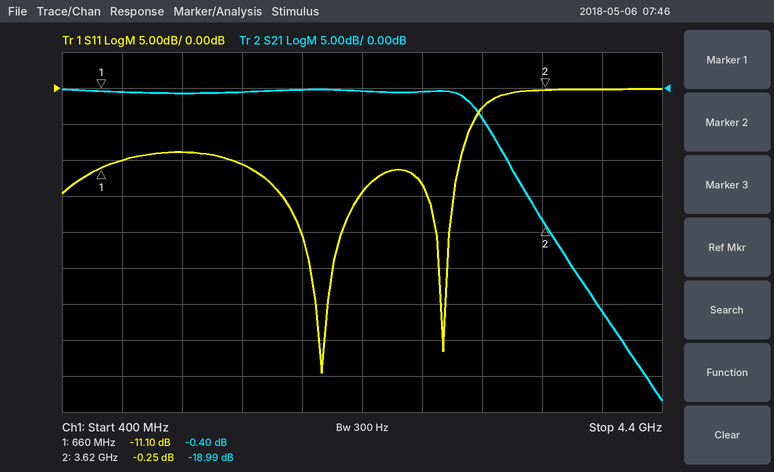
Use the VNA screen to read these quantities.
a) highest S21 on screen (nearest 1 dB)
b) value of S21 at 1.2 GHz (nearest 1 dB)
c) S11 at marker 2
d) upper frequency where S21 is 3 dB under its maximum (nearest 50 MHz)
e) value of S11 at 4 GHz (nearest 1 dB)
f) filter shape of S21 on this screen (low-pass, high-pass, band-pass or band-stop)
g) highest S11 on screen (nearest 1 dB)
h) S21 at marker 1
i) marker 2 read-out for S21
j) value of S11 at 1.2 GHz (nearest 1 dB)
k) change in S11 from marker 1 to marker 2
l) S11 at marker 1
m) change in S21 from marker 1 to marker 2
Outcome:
0 dB
-1 dB
-0.25 dB
3.15 GHz
0 dB
low-pass
0 dB
-0.40 dB
-18.99 dB
-9 dB
10.85 dB
-11.10 dB
-18.59 dB
